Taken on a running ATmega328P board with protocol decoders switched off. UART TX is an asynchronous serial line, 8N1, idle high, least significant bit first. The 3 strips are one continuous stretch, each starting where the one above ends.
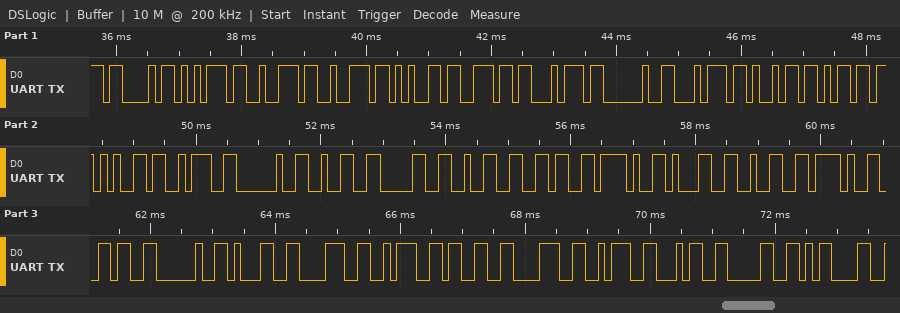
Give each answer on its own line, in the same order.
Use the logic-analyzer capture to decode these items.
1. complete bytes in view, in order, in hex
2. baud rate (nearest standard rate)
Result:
43 75 72 72 65 6E 74 20 74 69 6D 65 3A 20 32 30 32 36 2F 31 32 2F 36 20 31 38 3A 33 38 3A 34 30 0D
9600 baud
